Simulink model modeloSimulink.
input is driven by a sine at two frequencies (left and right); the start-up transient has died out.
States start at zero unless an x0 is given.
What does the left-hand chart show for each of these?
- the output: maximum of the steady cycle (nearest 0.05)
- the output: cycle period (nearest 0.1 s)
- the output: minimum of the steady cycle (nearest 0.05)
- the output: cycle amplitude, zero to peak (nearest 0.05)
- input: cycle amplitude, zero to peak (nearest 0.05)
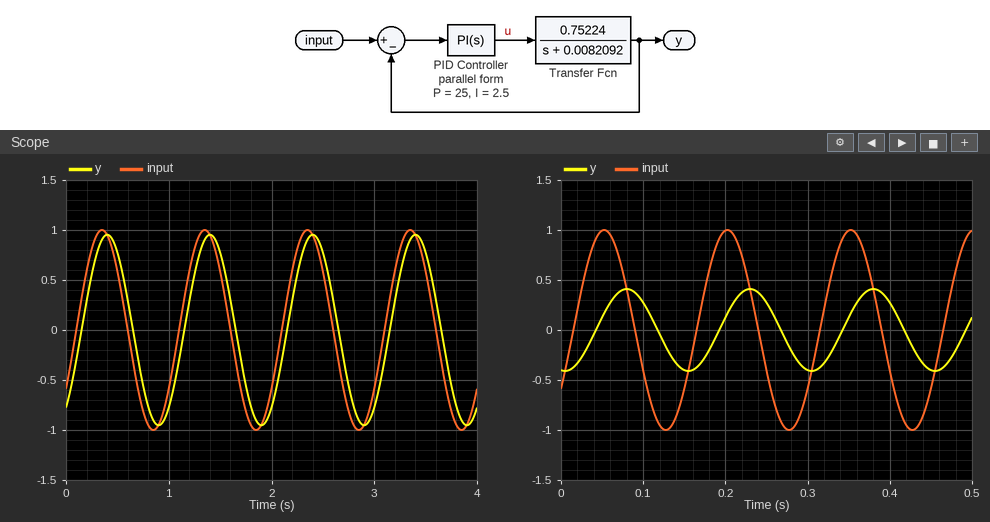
0.95
1.0 s
-0.95
0.95
1.00
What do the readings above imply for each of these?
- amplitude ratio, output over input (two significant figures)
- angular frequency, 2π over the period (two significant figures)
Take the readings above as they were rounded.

0.95
6.3 rad/s
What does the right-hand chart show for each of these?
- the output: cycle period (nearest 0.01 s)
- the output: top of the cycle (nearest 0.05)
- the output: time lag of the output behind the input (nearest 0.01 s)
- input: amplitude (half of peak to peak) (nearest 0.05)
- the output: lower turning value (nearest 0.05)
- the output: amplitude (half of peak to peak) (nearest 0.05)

0.15 s
0.40
0.03 s
1.00
-0.40
0.40
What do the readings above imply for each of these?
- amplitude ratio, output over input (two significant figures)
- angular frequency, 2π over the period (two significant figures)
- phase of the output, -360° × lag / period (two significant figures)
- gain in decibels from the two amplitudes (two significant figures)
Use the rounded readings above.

0.40
42 rad/s
-72°
-8.0 dB
